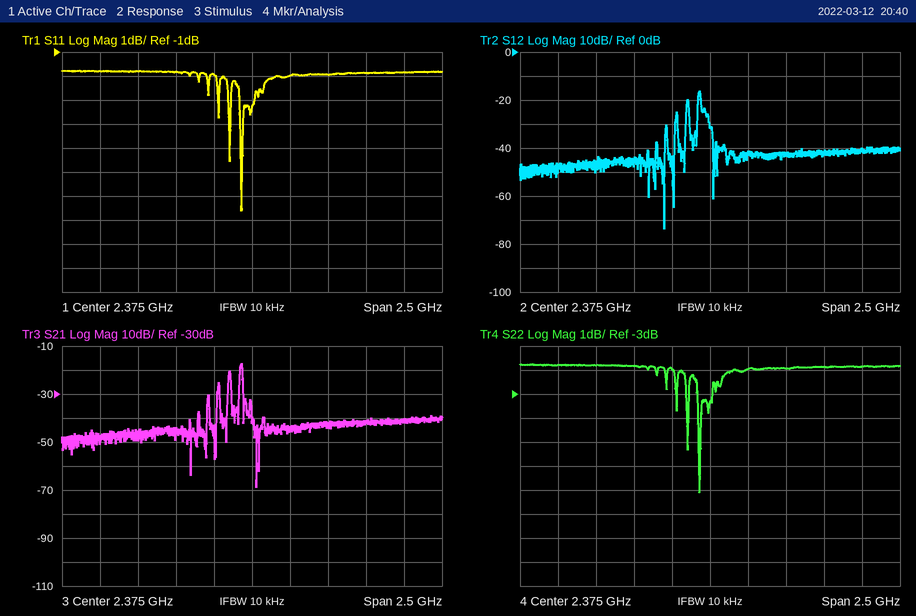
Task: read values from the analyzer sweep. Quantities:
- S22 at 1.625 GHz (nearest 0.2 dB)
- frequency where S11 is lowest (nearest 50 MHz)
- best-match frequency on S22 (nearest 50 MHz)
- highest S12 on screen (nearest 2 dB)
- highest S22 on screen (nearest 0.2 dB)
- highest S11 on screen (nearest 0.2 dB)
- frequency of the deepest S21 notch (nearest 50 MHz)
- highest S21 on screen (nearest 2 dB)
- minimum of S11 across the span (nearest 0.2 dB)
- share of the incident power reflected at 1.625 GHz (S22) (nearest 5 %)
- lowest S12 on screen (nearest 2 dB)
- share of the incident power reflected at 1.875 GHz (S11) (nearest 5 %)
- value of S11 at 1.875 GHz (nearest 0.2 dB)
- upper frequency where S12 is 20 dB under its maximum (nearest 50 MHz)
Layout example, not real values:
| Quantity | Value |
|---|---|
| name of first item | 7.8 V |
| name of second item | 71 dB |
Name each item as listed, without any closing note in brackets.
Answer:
| Quantity | Value |
|---|---|
| S22 at 1.625 GHz | -1.8 dB |
| frequency where S11 is lowest | 2.30 GHz |
| best-match frequency on S22 | 2.30 GHz |
| highest S12 on screen | -16 dB |
| highest S22 on screen | -1.8 dB |
| highest S11 on screen | -1.8 dB |
| frequency of the deepest S21 notch | 2.40 GHz |
| highest S21 on screen | -18 dB |
| minimum of S11 across the span | -7.6 dB |
| share of the incident power reflected at 1.625 GHz (S22) | 65 % |
| lowest S12 on screen | -74 dB |
| share of the incident power reflected at 1.875 GHz (S11) | 65 % |
| value of S11 at 1.875 GHz | -1.8 dB |
| upper frequency where S12 is 20 dB under its maximum | 2.40 GHz |
